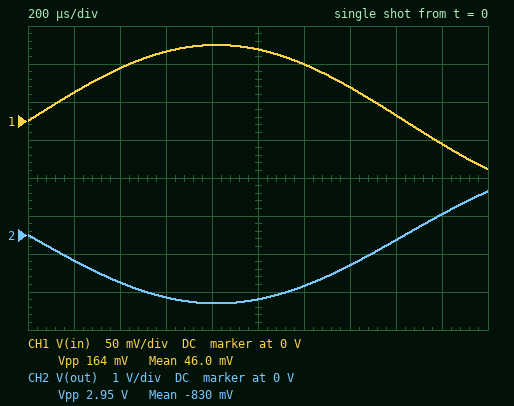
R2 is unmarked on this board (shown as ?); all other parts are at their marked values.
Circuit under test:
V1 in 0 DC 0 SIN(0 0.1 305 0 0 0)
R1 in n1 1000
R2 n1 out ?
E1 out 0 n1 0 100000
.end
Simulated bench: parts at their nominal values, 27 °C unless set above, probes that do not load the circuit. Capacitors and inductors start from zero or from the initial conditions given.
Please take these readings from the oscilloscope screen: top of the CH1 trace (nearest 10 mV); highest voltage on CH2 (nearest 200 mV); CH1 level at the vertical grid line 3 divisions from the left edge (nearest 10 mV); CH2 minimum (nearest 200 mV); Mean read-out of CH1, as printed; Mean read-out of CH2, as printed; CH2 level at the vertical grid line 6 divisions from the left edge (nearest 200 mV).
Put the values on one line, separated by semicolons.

100 mV; 1.2 V; 90 mV; -1.8 V; 46.0 mV; -830 mV; -1.4 V
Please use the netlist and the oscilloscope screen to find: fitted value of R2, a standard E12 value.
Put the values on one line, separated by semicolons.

18 kΩ
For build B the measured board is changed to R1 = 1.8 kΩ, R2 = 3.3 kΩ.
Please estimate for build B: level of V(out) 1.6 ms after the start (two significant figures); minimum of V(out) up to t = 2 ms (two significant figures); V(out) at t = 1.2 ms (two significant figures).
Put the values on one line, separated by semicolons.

-14 mV; -180 mV; -140 mV
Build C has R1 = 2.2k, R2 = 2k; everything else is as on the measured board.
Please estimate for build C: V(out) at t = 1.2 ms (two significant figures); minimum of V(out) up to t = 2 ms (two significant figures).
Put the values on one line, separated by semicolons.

-68 mV; -91 mV
